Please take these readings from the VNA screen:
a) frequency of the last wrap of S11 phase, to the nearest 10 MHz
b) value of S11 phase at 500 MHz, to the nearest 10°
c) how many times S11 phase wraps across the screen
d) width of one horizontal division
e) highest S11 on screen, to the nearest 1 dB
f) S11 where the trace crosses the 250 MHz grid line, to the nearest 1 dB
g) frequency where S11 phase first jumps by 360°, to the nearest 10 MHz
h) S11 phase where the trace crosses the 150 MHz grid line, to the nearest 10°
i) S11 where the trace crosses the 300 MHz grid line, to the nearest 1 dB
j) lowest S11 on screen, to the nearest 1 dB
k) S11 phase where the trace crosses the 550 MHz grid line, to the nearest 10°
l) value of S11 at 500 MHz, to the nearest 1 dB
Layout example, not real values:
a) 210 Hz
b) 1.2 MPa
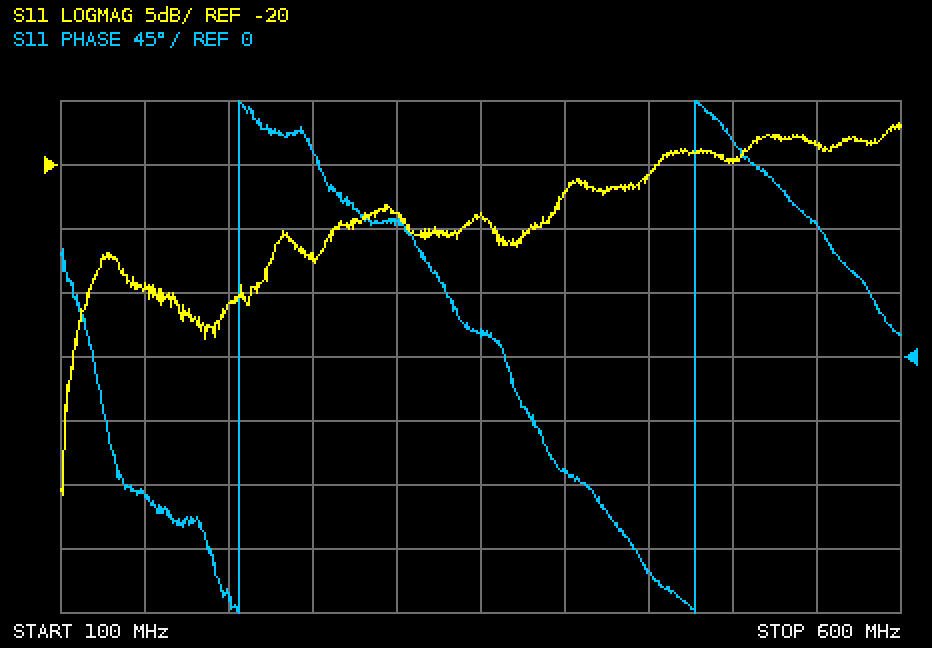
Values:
a) 480 MHz
b) 150°
c) 2
d) 50 MHz
e) -17 dB
f) -27 dB
g) 210 MHz
h) -100°
i) -24 dB
j) -46 dB
k) 90°
l) -20 dB
